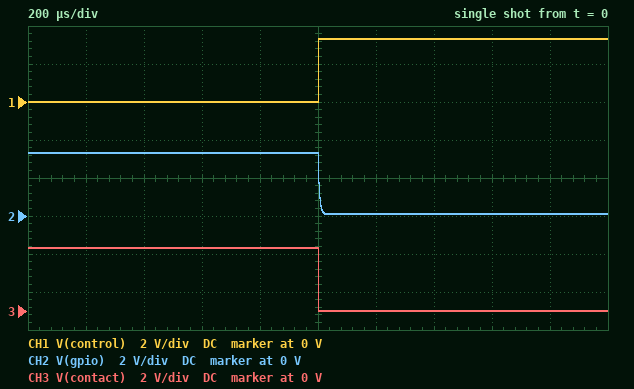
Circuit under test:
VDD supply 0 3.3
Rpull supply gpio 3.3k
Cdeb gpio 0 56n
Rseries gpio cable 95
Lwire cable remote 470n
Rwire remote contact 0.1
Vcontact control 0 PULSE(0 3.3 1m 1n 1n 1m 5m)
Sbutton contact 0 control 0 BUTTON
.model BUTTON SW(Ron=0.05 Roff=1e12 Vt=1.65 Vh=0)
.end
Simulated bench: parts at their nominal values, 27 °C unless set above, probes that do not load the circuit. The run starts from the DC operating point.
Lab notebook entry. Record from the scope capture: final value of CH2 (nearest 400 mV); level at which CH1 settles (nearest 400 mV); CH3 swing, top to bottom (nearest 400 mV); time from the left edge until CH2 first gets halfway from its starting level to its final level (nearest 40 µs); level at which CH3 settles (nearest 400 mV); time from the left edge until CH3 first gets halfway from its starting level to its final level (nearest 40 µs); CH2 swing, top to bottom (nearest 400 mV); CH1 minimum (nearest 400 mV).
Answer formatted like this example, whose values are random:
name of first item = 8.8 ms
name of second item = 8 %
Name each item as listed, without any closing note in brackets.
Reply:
final value of CH2 = 0 V
level at which CH1 settles = 3.2 V
CH3 swing, top to bottom = 3.2 V
time from the left edge until CH2 first gets halfway from its starting level to its final level = 1.00 ms
level at which CH3 settles = 0 V
time from the left edge until CH3 first gets halfway from its starting level to its final level = 1.00 ms
CH2 swing, top to bottom = 3.2 V
CH1 minimum = 0 V
